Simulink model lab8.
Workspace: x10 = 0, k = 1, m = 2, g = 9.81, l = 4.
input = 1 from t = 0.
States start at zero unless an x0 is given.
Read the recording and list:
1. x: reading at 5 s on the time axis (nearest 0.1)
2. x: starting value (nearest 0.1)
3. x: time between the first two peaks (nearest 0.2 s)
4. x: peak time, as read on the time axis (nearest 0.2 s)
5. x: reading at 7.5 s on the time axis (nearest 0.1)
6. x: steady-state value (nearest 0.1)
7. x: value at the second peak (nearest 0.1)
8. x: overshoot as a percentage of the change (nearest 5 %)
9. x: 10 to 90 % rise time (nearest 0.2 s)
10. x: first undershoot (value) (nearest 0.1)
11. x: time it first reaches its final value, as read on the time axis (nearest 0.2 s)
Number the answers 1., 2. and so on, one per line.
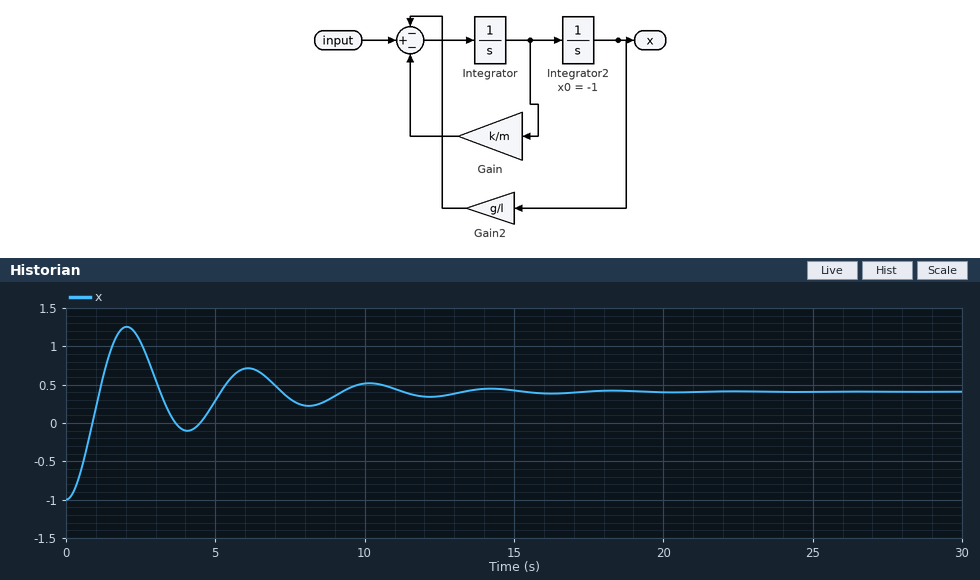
1. 0.3
2. -1.0
3. 4.0 s
4. 2.0 s
5. 0.3
6. 0.4
7. 0.7
8. 60 %
9. 0.8 s
10. -0.1
11. 1.2 s
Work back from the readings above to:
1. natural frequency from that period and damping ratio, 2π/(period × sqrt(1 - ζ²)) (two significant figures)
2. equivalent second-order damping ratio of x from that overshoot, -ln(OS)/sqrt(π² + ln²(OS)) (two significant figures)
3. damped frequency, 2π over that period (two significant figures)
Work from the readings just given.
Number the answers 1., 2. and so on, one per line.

1. 1.6 rad/s
2. 0.16
3. 1.6 rad/s
